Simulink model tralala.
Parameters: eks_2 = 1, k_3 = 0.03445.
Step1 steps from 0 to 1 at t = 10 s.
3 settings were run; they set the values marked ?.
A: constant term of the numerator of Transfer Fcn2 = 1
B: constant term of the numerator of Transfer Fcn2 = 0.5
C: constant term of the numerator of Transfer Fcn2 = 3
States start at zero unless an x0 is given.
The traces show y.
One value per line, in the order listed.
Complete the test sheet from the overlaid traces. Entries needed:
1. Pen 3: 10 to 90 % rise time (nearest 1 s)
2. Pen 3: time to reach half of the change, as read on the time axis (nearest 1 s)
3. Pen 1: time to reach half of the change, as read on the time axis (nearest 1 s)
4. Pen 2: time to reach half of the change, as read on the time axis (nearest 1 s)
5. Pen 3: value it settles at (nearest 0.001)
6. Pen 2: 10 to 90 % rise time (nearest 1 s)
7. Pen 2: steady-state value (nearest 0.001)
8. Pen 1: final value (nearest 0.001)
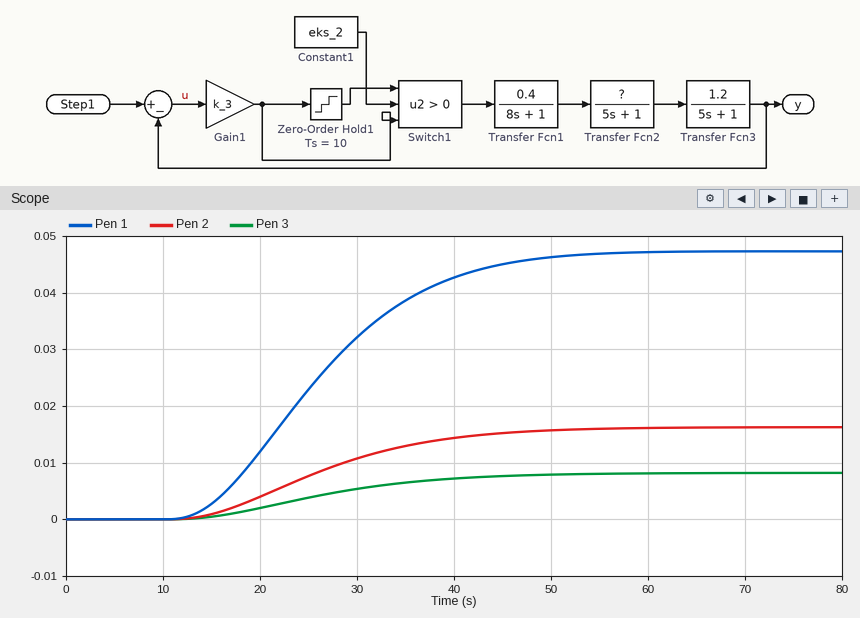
25 s
26 s
25 s
26 s
0.008
25 s
0.016
0.047
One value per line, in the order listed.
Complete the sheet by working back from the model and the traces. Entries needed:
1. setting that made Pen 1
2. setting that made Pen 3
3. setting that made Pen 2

C
B
A
